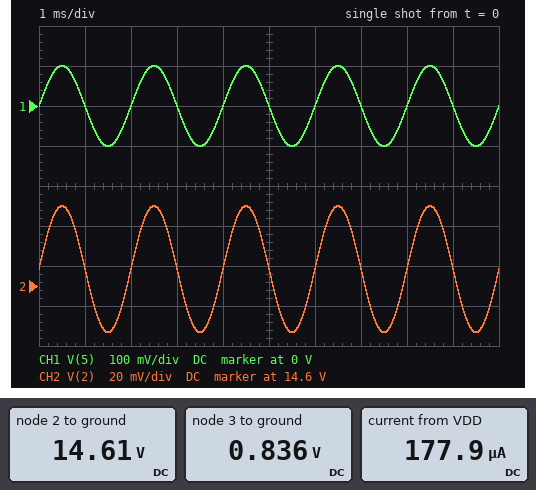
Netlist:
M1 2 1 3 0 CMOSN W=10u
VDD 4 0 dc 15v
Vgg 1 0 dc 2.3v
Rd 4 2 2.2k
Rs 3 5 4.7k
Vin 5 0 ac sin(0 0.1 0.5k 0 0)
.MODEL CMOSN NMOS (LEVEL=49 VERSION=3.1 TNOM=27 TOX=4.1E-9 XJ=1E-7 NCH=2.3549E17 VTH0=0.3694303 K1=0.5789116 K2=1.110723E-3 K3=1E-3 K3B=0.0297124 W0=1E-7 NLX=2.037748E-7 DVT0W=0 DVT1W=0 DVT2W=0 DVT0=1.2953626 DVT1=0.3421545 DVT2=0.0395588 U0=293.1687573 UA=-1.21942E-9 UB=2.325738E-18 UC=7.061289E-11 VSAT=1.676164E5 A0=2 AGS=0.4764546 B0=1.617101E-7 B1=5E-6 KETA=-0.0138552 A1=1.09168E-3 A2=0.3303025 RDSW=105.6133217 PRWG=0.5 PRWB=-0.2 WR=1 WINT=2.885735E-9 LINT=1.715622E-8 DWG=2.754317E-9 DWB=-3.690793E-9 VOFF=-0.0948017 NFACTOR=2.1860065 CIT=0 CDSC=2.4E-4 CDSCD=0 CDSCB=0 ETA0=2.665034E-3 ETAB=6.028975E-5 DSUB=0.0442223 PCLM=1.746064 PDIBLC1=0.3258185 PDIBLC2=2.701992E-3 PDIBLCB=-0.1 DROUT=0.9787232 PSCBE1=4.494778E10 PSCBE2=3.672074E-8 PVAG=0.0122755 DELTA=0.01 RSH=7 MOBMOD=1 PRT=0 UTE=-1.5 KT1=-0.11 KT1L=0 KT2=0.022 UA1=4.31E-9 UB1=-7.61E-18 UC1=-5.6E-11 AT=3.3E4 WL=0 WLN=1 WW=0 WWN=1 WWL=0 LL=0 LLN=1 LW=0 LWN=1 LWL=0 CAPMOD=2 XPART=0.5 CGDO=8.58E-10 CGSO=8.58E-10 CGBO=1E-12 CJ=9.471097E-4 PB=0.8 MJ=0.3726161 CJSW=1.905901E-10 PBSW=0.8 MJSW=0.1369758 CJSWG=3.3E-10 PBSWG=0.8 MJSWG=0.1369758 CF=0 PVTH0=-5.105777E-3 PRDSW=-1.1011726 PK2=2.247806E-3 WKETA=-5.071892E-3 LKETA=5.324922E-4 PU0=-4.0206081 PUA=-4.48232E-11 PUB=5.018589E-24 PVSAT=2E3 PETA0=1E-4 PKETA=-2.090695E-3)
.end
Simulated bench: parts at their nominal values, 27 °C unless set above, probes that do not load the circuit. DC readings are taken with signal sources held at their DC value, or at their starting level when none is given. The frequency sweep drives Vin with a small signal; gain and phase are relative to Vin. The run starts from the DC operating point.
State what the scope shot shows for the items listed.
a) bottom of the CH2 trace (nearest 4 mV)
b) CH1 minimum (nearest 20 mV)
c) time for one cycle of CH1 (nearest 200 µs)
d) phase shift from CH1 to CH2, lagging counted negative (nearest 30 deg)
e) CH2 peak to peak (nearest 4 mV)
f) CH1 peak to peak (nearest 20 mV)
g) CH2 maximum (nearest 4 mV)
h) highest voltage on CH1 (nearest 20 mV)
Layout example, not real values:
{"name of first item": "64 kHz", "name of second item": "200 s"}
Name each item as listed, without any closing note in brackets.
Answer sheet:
{"bottom of the CH2 trace": "14.576 V", "CH1 minimum": "-100 mV", "time for one cycle of CH1": "2.0 ms", "phase shift from CH1 to CH2, lagging counted negative": "0 deg", "CH2 peak to peak": "64 mV", "CH1 peak to peak": "200 mV", "CH2 maximum": "14.640 V", "highest voltage on CH1": "100 mV"}
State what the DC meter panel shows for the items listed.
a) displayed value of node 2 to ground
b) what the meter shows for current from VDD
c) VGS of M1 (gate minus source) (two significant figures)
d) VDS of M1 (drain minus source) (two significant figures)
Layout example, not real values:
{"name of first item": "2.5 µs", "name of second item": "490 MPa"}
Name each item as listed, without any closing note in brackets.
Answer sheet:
{"displayed value of node 2 to ground": "14.61 V", "what the meter shows for current from VDD": "177.9 µA", "VGS of M1 (gate minus source)": "1.5 V", "VDS of M1 (drain minus source)": "14 V"}
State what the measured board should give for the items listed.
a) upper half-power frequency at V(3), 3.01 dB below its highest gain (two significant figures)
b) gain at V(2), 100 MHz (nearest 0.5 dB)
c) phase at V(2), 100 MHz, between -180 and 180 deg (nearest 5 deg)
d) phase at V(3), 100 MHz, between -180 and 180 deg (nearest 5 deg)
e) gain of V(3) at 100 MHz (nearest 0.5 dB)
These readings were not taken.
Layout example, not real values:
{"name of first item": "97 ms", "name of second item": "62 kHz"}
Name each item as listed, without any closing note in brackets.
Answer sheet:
{"upper half-power frequency at V(3), 3.01 dB below its highest gain": "570 MHz", "gain at V(2), 100 MHz": "-10.0 dB", "phase at V(2), 100 MHz, between -180 and 180 deg": "-25 deg", "phase at V(3), 100 MHz, between -180 and 180 deg": "-10 deg", "gain of V(3) at 100 MHz": "-10.0 dB"}
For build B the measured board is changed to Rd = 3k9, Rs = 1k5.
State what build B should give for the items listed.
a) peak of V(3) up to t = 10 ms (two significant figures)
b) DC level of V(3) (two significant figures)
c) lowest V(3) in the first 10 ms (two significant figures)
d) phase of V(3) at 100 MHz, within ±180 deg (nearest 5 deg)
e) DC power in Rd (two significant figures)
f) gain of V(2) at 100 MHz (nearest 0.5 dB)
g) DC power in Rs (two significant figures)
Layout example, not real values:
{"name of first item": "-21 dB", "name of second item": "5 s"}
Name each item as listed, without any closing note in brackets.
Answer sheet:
{"peak of V(3) up to t = 10 ms": "570 mV", "DC level of V(3)": "510 mV", "lowest V(3) in the first 10 ms": "460 mV", "phase of V(3) at 100 MHz, within ±180 deg": "-5 deg", "DC power in Rd": "460 µW", "gain of V(2) at 100 MHz": "2.0 dB", "DC power in Rs": "180 µW"}
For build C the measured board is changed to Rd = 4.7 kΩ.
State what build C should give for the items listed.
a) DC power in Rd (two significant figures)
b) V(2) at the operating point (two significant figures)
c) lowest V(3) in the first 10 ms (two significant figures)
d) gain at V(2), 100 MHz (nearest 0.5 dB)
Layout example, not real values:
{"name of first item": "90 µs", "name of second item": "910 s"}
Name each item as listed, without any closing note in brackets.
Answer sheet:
{"DC power in Rd": "150 µW", "V(2) at the operating point": "14 V", "lowest V(3) in the first 10 ms": "800 mV", "gain at V(2), 100 MHz": "-3.5 dB"}
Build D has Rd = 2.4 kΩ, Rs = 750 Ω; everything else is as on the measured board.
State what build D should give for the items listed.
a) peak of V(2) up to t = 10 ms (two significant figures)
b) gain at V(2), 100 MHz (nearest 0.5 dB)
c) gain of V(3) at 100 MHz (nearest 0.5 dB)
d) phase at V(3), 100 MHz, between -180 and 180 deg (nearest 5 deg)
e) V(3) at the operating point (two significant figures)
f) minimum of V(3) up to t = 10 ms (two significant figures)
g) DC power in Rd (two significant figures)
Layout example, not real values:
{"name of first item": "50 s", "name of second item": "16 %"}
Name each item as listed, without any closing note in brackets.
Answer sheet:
{"peak of V(2) up to t = 10 ms": "14 V", "gain at V(2), 100 MHz": "0.5 dB", "gain of V(3) at 100 MHz": "-3.5 dB", "phase at V(3), 100 MHz, between -180 and 180 deg": "-5 deg", "V(3) at the operating point": "340 mV", "minimum of V(3) up to t = 10 ms": "270 mV", "DC power in Rd": "490 µW"}
